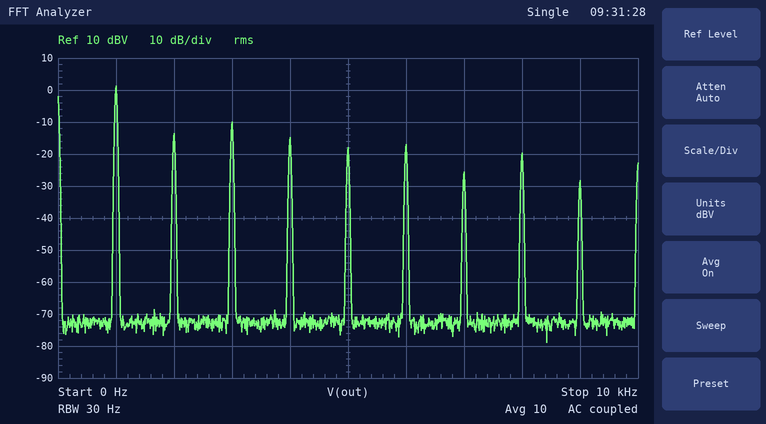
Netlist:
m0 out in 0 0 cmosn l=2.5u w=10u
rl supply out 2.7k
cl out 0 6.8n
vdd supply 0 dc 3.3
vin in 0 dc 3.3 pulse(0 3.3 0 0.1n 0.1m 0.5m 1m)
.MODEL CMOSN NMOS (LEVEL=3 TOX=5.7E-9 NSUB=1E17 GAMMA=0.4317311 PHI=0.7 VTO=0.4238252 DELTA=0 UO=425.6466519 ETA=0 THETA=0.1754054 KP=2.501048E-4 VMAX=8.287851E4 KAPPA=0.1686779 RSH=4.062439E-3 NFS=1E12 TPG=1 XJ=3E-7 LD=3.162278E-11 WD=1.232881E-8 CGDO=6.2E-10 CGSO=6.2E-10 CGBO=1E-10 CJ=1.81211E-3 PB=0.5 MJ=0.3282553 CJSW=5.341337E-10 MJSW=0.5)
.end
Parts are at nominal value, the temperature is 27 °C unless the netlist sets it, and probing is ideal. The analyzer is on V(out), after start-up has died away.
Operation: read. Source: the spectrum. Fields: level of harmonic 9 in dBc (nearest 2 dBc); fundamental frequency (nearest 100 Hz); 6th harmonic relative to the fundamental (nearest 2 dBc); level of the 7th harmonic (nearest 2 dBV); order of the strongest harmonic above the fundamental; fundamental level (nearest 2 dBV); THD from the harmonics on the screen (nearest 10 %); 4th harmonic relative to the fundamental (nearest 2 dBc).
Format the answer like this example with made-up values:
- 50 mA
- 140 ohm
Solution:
- -30 dBc
- 1.0 kHz
- -18 dBc
- -26 dBV
- 3
- 2 dBV
- 40 %
- -16 dBc
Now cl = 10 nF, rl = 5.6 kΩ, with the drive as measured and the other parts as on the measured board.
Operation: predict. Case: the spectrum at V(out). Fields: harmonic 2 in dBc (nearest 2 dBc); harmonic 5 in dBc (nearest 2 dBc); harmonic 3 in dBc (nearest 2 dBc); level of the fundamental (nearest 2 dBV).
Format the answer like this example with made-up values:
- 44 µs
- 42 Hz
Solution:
- -12 dBc
- -22 dBc
- -14 dBc
- 2 dBV
